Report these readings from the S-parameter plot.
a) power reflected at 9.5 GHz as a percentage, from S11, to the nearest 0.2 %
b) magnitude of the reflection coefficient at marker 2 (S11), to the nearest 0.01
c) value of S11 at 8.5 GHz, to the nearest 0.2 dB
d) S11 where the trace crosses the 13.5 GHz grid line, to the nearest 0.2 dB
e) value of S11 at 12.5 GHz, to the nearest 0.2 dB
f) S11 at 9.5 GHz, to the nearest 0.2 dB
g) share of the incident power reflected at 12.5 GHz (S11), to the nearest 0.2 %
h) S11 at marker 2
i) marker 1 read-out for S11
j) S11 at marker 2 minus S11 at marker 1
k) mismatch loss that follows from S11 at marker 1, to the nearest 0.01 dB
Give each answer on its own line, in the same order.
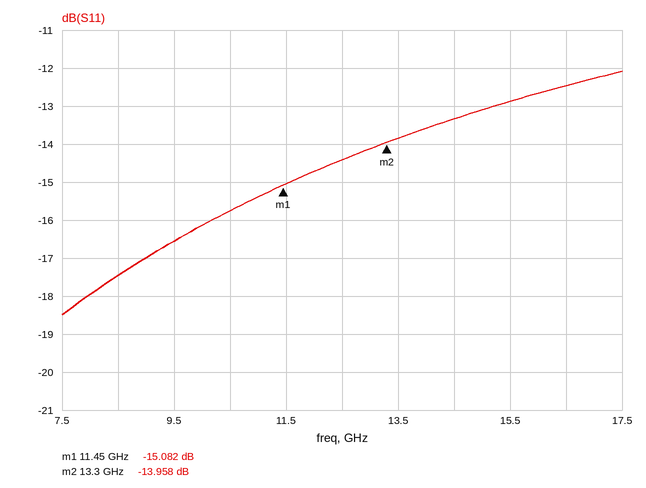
2.2 %
0.20
-17.4 dB
-13.8 dB
-14.4 dB
-16.6 dB
3.6 %
-13.958 dB
-15.082 dB
1.124 dB
0.14 dB
